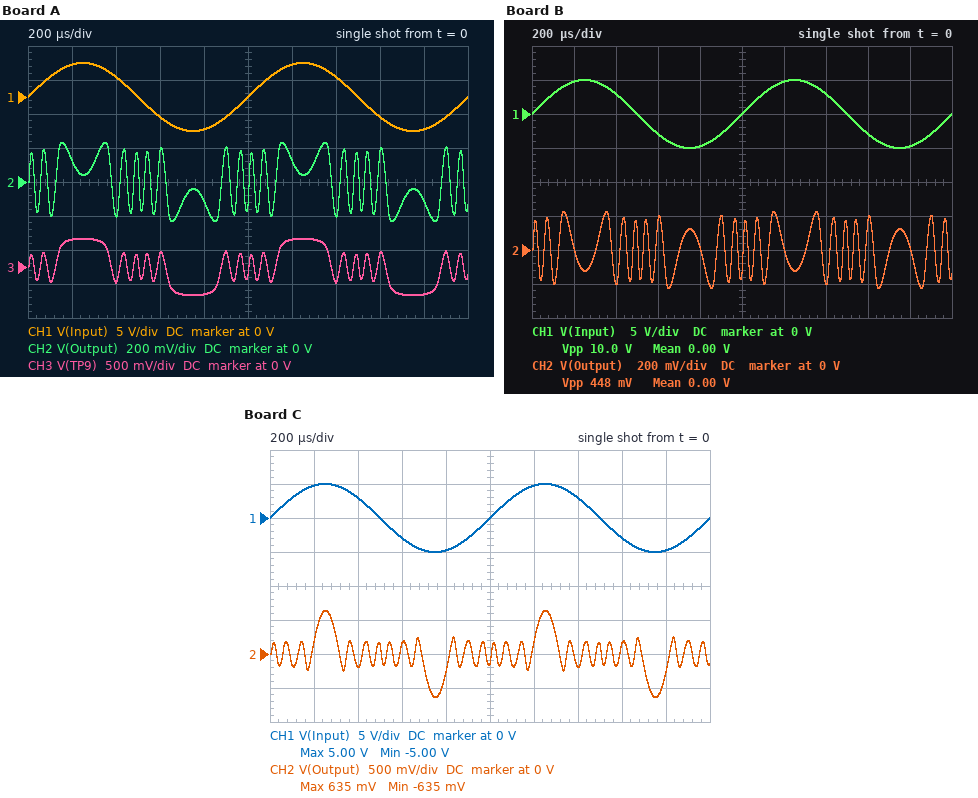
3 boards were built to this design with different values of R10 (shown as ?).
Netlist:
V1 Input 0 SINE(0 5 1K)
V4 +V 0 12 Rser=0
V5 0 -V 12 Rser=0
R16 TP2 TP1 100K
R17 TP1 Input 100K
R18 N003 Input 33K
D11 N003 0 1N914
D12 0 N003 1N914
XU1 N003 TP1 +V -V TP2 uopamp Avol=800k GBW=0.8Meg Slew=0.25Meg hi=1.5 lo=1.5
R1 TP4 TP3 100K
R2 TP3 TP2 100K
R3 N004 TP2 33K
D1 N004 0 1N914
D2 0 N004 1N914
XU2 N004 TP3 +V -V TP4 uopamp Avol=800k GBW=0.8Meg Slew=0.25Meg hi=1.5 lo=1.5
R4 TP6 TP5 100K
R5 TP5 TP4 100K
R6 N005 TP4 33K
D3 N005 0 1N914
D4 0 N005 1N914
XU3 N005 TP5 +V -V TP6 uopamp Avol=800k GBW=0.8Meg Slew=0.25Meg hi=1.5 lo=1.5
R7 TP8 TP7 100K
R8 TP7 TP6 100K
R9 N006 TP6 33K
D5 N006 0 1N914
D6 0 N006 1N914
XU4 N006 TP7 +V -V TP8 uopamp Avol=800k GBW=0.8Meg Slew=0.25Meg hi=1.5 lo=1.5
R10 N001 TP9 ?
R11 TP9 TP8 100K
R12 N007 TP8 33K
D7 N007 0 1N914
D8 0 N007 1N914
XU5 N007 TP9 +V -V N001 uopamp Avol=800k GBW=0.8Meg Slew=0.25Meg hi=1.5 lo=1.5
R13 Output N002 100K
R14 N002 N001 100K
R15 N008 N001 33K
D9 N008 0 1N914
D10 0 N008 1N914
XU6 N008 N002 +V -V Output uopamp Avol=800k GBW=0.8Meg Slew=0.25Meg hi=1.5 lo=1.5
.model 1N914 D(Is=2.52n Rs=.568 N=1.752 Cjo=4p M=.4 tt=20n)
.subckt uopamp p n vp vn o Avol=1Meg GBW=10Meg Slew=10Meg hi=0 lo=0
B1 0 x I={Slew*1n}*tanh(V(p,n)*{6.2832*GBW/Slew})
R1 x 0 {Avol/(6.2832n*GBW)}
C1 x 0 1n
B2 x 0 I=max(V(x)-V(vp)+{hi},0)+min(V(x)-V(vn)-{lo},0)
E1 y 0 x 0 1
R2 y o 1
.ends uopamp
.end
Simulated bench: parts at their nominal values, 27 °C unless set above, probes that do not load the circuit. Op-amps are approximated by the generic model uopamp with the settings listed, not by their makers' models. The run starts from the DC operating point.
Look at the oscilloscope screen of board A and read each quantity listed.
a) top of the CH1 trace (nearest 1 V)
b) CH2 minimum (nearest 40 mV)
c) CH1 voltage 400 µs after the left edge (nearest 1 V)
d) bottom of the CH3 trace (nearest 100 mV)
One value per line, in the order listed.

5 V
-240 mV
3 V
-400 mV
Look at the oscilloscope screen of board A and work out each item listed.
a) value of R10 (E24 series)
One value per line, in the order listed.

47 kΩ
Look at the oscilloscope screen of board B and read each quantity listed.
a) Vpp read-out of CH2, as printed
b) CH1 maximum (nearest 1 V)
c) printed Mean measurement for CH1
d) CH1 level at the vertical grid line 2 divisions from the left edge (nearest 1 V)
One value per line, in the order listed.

448 mV
5 V
0.00 V
3 V
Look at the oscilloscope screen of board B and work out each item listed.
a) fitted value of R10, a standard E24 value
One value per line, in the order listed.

68 kΩ
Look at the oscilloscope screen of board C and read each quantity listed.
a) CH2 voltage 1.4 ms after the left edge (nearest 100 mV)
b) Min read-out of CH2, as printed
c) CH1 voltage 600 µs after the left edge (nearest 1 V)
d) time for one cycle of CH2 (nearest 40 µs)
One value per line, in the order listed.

-200 mV
-635 mV
-3 V
1.00 ms
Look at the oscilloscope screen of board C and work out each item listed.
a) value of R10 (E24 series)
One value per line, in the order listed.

240 kΩ
